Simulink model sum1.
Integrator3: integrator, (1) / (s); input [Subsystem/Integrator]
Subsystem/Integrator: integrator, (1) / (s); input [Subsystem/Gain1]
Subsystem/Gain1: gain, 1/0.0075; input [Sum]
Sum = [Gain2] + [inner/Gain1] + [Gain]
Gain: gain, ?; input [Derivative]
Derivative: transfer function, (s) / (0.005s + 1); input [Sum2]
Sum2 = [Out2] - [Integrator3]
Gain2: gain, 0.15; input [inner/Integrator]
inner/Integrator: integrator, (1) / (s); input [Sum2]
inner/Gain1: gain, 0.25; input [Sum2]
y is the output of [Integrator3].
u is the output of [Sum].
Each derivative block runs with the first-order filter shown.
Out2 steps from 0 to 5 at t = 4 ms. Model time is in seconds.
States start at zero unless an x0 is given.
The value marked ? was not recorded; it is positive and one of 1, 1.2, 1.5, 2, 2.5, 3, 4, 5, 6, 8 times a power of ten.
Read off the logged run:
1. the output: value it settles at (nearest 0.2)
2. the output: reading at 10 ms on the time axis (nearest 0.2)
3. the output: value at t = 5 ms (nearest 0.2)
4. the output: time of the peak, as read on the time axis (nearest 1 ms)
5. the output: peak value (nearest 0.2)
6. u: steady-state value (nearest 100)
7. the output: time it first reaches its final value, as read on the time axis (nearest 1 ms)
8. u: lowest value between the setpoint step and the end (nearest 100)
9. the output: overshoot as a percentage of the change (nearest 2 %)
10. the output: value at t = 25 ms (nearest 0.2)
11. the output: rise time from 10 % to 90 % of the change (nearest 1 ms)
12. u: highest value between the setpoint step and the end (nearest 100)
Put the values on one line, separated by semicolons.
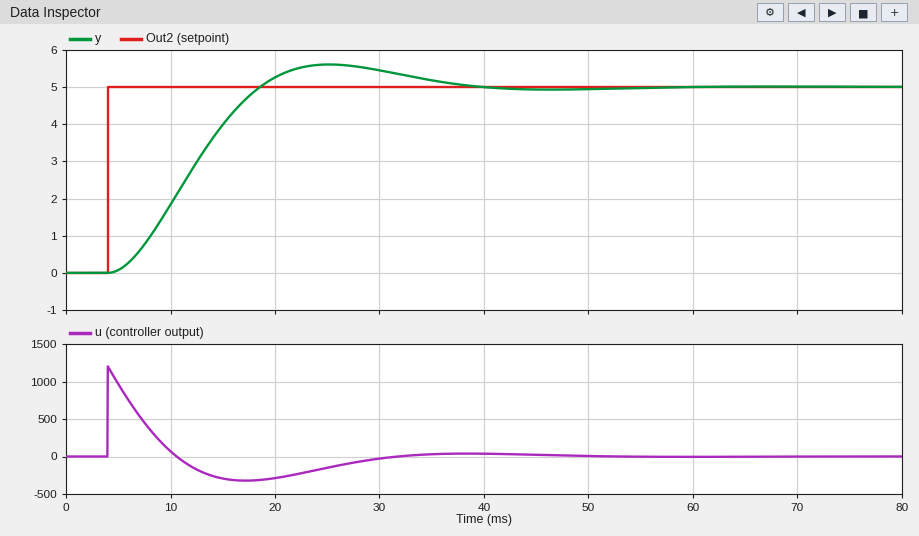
5.0; 1.8; 0.0; 25 ms; 5.6; 0; 19 ms; -300; 12 %; 5.6; 10 ms; 1200
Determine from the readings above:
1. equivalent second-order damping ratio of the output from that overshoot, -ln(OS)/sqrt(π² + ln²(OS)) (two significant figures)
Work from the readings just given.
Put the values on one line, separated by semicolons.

0.56
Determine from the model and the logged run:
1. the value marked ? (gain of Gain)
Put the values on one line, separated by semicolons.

1.2
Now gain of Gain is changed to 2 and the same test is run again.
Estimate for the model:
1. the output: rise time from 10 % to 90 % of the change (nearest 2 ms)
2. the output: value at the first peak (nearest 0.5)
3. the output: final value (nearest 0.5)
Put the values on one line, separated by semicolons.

6 ms; 6.0; 5.0
